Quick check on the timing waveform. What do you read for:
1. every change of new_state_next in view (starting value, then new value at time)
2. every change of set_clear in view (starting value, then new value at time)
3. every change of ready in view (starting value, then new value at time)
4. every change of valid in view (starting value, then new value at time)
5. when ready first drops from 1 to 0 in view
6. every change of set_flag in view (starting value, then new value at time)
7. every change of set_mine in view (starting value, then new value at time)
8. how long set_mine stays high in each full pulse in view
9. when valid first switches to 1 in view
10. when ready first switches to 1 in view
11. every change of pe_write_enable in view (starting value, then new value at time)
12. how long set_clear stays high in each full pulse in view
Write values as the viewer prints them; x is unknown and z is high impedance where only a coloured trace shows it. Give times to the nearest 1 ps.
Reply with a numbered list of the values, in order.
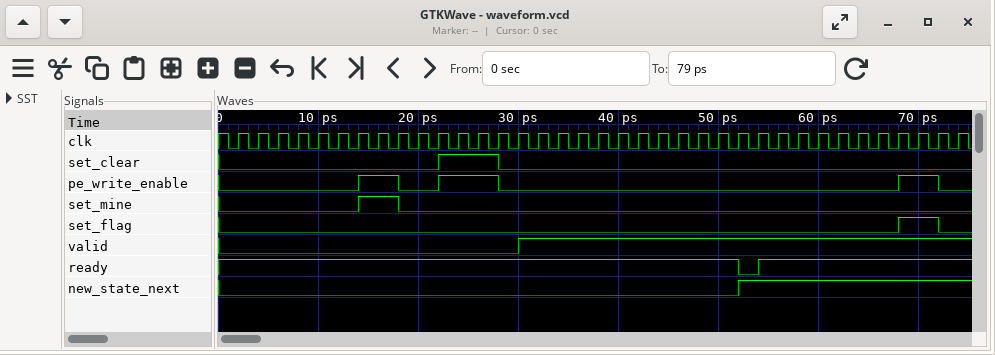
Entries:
1. 0, 1 at 52 ps
2. 0, 1 at 22 ps, 0 at 28 ps
3. 1, 0 at 52 ps, 1 at 54 ps
4. 0, 1 at 30 ps
5. 52 ps
6. 0, 1 at 68 ps, 0 at 72 ps
7. 0, 1 at 14 ps, 0 at 18 ps
8. 4 ps
9. 30 ps
10. 54 ps
11. 0, 1 at 14 ps, 0 at 18 ps, 1 at 22 ps, 0 at 28 ps, 1 at 68 ps, 0 at 72 ps
12. 6 ps
